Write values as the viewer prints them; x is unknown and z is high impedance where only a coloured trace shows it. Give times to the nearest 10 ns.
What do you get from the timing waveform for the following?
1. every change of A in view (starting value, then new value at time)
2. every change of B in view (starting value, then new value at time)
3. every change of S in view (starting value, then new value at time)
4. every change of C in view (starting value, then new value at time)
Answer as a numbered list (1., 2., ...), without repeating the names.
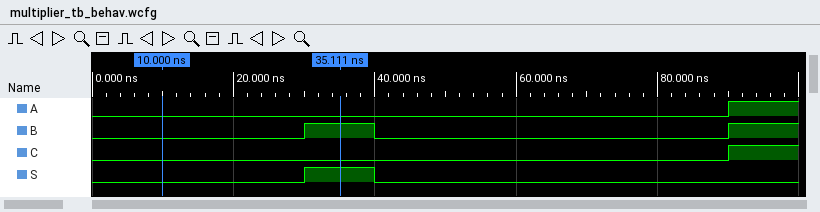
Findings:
1. 0, 1 at 90 ns
2. 0, 1 at 30 ns, 0 at 40 ns, 1 at 90 ns
3. 0, 1 at 30 ns, 0 at 40 ns
4. 0, 1 at 90 ns
